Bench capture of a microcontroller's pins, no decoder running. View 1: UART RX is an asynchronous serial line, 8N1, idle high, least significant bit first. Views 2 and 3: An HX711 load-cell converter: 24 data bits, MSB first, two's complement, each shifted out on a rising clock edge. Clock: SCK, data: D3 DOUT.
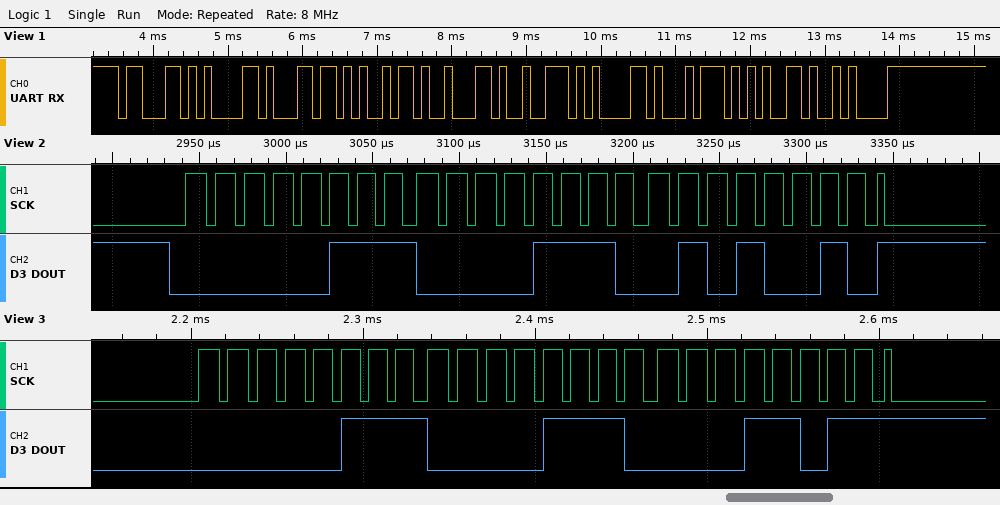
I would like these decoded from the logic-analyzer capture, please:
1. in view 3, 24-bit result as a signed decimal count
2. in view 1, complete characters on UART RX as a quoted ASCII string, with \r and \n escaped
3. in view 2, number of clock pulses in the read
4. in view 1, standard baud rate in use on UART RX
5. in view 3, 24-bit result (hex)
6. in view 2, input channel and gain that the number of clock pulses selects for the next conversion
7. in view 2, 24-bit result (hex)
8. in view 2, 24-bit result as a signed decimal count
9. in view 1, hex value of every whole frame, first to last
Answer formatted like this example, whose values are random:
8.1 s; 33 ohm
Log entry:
462363; "calibrate\n"; 25; 9600 baud; 0x070E1B; channel A, gain 128; 0x070E52; 462418; 63 61 6C 69 62 72 61 74 65 0A
